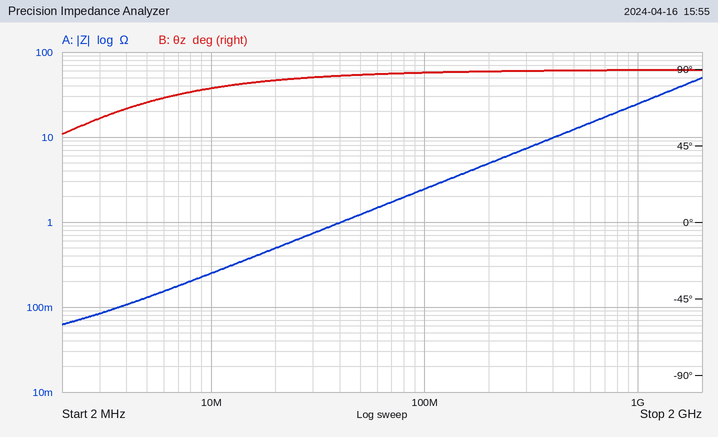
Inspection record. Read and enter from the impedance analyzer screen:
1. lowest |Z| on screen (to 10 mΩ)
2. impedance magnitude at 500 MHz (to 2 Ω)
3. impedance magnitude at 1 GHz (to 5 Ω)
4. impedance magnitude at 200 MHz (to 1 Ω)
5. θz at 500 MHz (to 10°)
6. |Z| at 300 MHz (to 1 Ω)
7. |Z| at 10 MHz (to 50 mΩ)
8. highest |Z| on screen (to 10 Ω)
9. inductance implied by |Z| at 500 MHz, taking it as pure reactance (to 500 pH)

60 mΩ
12 Ω
25 Ω
5 Ω
90°
7 Ω
250 mΩ
50 Ω
4.0 nH
